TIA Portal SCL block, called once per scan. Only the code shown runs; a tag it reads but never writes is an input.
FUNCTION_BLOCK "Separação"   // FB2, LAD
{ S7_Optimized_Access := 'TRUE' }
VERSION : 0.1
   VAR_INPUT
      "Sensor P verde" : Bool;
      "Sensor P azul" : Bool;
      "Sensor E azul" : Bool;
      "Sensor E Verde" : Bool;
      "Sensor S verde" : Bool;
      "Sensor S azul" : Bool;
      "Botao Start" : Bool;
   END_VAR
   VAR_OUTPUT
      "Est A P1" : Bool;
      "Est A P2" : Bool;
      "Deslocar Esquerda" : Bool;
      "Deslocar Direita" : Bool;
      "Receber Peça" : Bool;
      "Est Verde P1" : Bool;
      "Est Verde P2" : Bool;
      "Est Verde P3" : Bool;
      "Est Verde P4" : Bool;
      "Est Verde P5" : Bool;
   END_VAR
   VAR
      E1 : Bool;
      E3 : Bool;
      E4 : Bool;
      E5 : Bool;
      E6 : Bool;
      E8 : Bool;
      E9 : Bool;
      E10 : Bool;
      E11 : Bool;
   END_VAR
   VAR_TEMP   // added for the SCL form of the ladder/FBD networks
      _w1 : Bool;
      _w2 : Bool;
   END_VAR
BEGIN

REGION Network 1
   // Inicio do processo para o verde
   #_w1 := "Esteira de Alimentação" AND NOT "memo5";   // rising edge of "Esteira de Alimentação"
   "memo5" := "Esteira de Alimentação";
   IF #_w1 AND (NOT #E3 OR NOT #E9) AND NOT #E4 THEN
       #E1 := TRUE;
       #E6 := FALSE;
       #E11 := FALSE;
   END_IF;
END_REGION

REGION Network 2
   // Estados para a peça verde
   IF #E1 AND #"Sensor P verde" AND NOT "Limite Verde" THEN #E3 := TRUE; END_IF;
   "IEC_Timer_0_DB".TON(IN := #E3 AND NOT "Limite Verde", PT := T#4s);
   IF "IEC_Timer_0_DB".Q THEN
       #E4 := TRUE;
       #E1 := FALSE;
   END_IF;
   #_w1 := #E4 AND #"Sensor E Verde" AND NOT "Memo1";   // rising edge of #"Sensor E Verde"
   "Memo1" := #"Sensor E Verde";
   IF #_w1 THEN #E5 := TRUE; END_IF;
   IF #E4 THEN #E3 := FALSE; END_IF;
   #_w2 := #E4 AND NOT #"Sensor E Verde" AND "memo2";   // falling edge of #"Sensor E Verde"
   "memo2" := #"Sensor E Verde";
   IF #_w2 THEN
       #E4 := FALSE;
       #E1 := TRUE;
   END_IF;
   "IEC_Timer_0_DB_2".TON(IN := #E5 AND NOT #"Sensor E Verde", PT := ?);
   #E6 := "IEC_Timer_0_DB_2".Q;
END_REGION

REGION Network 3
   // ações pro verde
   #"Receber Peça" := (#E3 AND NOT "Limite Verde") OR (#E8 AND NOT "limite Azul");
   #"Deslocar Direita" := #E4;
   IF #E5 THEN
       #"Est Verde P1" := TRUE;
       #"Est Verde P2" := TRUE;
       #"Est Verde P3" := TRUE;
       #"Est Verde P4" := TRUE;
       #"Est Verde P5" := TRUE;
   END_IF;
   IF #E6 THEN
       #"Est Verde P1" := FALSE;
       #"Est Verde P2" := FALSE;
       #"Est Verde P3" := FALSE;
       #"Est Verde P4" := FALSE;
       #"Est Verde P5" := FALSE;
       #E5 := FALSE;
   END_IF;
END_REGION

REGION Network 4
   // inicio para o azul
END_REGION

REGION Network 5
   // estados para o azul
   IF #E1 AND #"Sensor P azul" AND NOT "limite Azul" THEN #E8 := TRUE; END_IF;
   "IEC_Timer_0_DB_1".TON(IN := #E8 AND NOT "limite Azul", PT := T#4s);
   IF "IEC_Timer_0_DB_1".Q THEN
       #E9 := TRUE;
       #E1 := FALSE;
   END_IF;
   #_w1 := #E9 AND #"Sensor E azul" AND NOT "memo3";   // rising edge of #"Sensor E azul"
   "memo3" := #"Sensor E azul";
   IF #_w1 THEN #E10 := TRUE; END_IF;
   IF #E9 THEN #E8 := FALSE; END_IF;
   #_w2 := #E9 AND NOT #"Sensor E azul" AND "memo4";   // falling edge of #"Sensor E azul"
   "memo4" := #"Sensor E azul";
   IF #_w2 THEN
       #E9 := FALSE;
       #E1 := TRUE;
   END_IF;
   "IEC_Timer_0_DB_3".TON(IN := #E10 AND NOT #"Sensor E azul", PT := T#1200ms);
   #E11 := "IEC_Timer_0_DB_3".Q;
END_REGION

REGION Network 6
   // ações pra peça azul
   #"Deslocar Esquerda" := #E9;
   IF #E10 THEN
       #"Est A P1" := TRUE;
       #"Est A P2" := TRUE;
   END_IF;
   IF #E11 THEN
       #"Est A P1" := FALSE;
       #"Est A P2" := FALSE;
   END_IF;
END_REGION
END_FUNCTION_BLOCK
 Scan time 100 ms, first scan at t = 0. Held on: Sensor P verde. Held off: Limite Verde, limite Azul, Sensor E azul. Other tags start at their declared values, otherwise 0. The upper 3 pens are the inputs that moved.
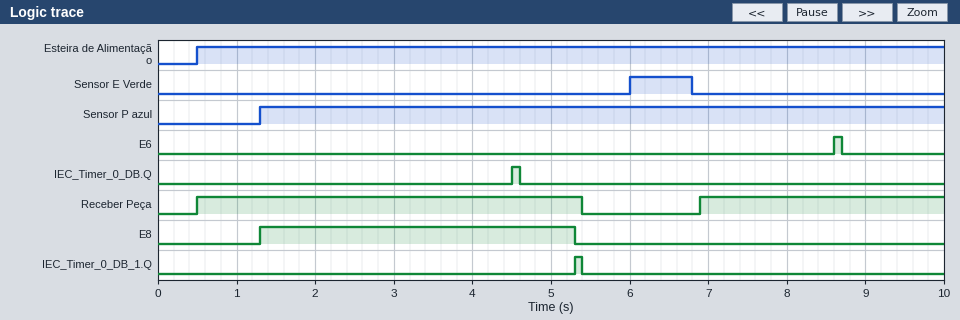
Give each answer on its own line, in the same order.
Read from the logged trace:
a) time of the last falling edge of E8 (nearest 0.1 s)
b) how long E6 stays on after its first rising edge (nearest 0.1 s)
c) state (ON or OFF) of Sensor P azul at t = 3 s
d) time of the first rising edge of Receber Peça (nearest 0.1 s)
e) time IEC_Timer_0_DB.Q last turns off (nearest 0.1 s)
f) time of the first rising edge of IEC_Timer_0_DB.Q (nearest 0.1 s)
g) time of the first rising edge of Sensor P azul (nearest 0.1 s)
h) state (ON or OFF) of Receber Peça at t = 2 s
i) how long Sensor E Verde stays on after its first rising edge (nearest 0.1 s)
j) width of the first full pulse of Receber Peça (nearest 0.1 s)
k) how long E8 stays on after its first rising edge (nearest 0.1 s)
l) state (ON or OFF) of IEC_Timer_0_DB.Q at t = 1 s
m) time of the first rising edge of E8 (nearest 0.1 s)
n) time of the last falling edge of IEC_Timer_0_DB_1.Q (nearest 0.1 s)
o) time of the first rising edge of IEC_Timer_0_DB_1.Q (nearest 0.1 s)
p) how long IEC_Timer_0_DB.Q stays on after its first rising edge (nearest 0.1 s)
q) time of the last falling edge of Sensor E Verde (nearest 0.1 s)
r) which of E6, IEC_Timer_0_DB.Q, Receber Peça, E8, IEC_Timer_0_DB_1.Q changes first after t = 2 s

5.3 s
0.1 s
ON
0.5 s
4.6 s
4.5 s
1.3 s
ON
0.8 s
4.9 s
4.0 s
OFF
1.3 s
5.4 s
5.3 s
0.1 s
6.8 s
IEC_Timer_0_DB.Q
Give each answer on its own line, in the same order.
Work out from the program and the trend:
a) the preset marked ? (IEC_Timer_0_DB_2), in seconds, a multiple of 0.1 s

1.8 s
